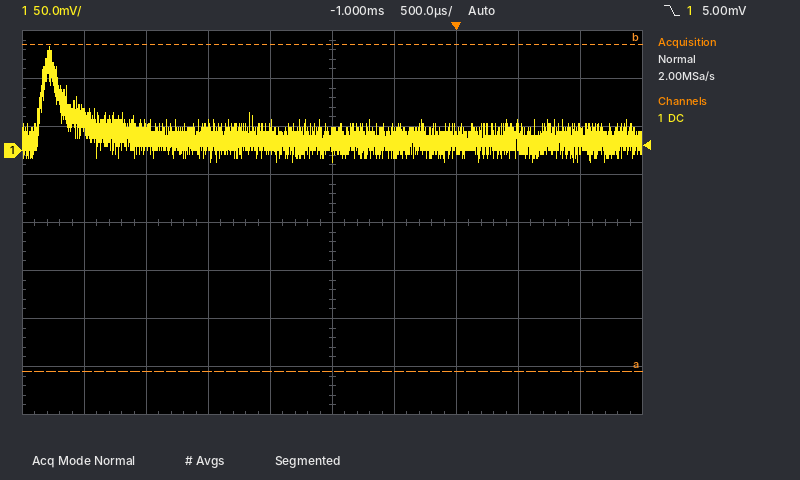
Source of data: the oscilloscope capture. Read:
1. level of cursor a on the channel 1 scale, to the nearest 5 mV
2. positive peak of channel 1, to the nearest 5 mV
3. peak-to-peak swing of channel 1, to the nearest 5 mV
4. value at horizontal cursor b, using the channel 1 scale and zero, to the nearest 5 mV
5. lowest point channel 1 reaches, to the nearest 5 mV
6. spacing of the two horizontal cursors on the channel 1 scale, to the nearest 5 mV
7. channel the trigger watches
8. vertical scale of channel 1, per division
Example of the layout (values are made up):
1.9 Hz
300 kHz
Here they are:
-230 mV
110 mV
120 mV
110 mV
-10 mV
340 mV
channel 1
50 mV
